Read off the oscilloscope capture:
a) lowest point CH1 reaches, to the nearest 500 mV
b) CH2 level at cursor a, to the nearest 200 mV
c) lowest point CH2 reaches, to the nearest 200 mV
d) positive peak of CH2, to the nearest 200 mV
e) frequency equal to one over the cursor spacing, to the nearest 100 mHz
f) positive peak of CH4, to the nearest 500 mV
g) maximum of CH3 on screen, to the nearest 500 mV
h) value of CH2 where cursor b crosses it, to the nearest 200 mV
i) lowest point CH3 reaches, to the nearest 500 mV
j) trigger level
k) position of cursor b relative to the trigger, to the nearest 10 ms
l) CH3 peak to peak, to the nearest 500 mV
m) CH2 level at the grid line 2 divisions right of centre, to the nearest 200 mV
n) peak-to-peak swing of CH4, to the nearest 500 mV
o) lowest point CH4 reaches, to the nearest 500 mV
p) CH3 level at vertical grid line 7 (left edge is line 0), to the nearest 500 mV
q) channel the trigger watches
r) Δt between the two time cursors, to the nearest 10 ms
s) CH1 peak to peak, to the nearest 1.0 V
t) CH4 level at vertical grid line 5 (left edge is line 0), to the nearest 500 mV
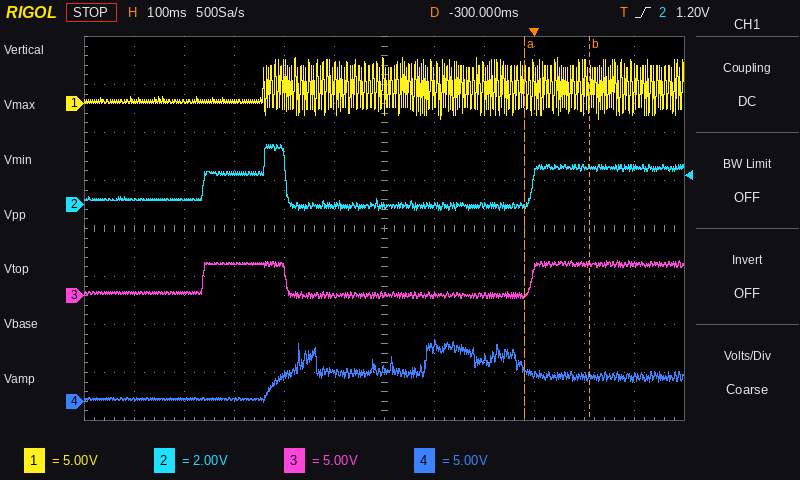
-1.5 V
0.0 V
-200 mV
2.4 V
7.7 Hz
6.5 V
3.5 V
1.6 V
-500 mV
1.20 V
+110 ms
4.0 V
0.0 V
6.5 V
0.0 V
0.0 V
CH2
130 ms
6.0 V
3.0 V
